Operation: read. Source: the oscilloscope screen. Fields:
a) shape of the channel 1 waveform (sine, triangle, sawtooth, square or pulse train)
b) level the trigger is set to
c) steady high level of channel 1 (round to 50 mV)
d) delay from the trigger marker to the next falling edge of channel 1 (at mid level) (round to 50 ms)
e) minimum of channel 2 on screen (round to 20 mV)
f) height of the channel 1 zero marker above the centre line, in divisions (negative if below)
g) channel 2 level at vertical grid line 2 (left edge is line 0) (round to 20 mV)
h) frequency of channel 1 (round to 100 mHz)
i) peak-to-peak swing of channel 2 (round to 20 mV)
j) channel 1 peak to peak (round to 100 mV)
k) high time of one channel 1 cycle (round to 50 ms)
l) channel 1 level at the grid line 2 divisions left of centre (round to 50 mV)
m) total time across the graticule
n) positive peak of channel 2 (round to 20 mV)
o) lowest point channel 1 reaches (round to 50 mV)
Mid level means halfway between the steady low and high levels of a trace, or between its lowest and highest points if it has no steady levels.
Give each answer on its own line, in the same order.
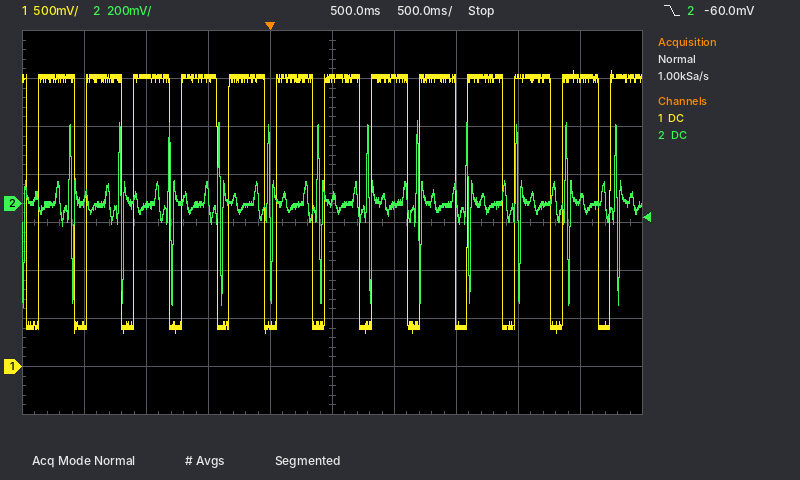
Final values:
pulse train
-60.0 mV
3.00 V
350 ms
-440 mV
-3.0 div
0 mV
2.6 Hz
780 mV
2.70 V
300 ms
3.00 V
5 s
340 mV
350 mV
